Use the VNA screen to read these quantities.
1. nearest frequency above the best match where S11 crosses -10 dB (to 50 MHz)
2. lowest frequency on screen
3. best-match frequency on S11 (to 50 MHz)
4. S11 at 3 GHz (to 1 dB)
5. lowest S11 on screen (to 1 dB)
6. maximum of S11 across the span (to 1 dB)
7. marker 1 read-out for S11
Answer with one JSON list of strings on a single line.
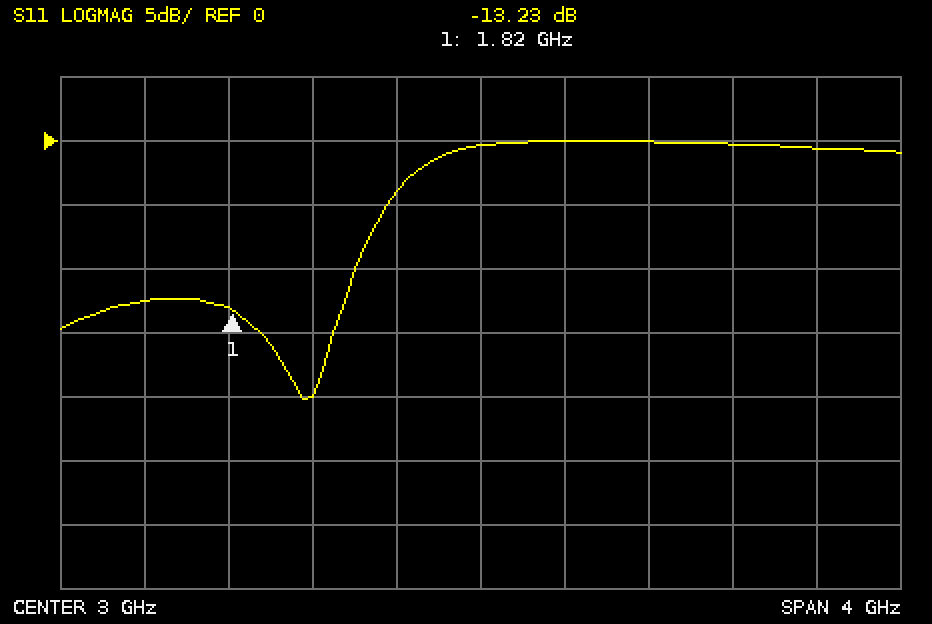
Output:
["2.40 GHz", "1 GHz", "2.15 GHz", "0 dB", "-20 dB", "0 dB", "-13.23 dB"]
